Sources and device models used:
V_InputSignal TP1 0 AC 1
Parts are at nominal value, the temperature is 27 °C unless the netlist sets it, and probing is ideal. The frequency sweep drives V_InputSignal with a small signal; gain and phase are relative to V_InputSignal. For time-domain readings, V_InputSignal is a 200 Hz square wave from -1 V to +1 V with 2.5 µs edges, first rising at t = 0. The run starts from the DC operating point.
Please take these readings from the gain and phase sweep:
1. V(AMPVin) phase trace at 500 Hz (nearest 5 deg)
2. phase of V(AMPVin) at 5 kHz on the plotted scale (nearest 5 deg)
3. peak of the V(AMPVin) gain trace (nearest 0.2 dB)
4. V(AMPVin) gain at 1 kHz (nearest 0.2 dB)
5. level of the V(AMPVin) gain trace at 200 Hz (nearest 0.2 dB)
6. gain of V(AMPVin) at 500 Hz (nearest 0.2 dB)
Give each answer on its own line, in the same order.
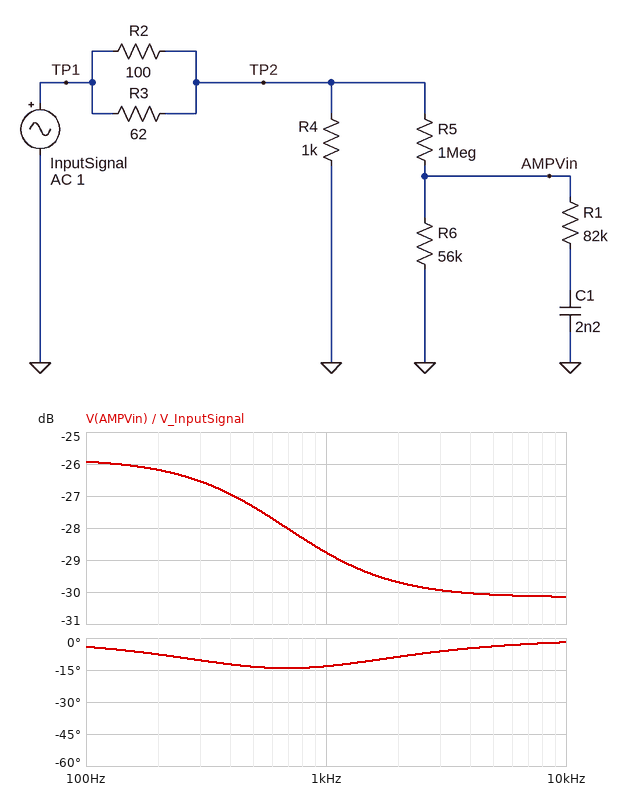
-15 deg
-5 deg
-26.0 dB
-28.8 dB
-26.2 dB
-27.4 dB
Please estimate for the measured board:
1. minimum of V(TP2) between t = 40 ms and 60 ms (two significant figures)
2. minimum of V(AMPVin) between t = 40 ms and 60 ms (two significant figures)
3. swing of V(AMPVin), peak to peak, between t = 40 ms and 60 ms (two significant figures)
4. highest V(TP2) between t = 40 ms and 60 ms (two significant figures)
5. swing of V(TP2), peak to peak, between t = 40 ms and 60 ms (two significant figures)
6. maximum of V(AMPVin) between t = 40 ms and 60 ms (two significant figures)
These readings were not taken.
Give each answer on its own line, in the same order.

-960 mV
-51 mV
100 mV
960 mV
1.9 V
51 mV
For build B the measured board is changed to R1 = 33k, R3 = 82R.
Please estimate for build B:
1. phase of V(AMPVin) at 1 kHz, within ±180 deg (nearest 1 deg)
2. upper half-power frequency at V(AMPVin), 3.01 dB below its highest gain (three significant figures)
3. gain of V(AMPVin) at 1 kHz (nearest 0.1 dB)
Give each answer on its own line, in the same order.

-25 deg
1.00 kHz
-28.9 dB
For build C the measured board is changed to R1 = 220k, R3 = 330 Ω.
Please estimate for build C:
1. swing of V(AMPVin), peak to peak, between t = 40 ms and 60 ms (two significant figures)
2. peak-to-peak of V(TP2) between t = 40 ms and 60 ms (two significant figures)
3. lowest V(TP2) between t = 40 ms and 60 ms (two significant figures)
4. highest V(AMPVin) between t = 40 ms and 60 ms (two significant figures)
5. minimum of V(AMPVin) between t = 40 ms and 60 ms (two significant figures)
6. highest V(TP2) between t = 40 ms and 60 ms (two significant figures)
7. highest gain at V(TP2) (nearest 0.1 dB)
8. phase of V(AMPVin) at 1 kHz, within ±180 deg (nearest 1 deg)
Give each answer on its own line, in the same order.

98 mV
1.9 V
-930 mV
49 mV
-49 mV
930 mV
-0.6 dB
-3 deg
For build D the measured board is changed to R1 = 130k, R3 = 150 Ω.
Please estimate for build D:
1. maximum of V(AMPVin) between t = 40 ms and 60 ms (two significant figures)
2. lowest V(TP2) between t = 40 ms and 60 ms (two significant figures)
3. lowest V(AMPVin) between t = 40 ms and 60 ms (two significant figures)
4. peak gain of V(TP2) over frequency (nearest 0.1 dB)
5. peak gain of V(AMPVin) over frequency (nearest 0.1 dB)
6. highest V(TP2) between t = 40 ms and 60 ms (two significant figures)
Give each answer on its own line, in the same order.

50 mV
-940 mV
-50 mV
-0.5 dB
-26.0 dB
940 mV
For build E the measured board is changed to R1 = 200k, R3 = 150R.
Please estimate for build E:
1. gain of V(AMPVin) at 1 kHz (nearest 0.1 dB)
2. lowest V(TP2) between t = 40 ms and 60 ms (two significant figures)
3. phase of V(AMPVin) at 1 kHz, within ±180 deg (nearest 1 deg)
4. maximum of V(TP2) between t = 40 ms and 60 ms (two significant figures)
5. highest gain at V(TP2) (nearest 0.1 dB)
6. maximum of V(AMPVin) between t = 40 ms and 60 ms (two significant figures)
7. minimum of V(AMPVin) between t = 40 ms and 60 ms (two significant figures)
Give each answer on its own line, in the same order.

-27.9 dB
-940 mV
-4 deg
940 mV
-0.5 dB
50 mV
-50 mV
